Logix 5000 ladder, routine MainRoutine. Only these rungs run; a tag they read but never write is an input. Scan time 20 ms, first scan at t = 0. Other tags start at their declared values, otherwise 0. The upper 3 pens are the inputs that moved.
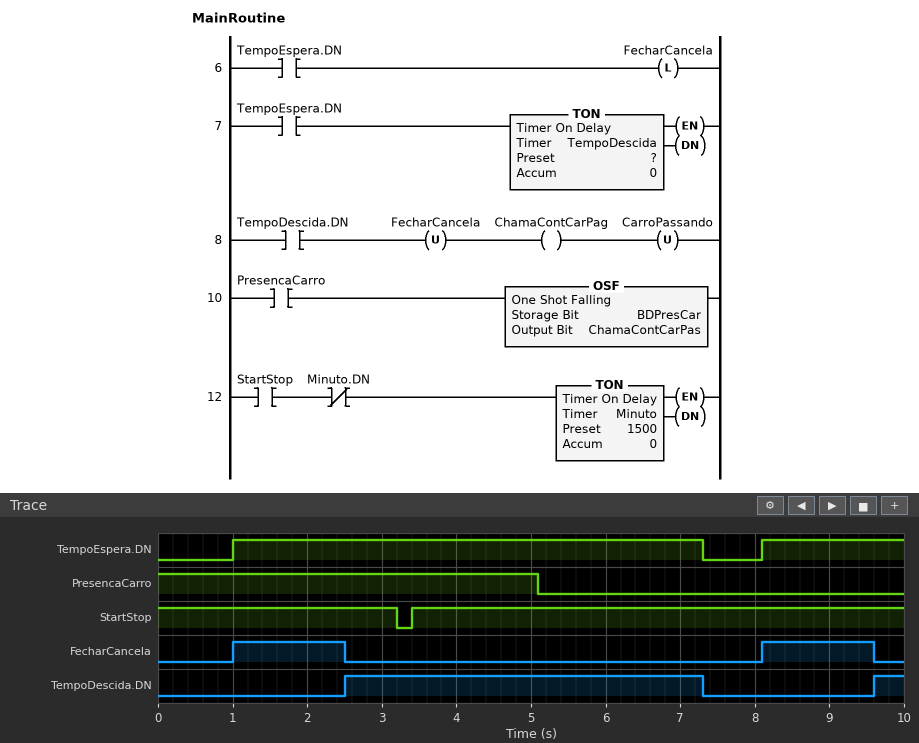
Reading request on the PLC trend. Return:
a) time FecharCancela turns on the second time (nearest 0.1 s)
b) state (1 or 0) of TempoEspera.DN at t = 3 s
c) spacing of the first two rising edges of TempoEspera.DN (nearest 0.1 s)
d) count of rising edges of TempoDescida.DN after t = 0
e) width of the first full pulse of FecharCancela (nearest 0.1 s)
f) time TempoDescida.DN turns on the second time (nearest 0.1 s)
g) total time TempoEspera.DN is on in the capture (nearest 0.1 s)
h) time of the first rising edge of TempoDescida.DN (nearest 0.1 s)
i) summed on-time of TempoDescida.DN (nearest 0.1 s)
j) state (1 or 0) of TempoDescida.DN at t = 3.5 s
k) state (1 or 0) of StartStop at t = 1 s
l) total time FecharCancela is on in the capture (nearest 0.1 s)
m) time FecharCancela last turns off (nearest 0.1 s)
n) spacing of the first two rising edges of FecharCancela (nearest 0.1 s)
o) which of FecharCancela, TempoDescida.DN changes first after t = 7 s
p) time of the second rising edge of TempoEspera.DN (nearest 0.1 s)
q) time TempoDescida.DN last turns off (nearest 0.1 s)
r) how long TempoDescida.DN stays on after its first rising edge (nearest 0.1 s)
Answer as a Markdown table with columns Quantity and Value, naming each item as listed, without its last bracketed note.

| Quantity | Value |
|---|---|
| time FecharCancela turns on the second time | 8.1 s |
| state (1 or 0) of TempoEspera.DN at t = 3 s | 1 |
| spacing of the first two rising edges of TempoEspera.DN | 7.1 s |
| count of rising edges of TempoDescida.DN after t = 0 | 2 |
| width of the first full pulse of FecharCancela | 1.5 s |
| time TempoDescida.DN turns on the second time | 9.6 s |
| total time TempoEspera.DN is on in the capture | 8.2 s |
| time of the first rising edge of TempoDescida.DN | 2.5 s |
| summed on-time of TempoDescida.DN | 5.2 s |
| state (1 or 0) of TempoDescida.DN at t = 3.5 s | 1 |
| state (1 or 0) of StartStop at t = 1 s | 1 |
| total time FecharCancela is on in the capture | 3.0 s |
| time FecharCancela last turns off | 9.6 s |
| spacing of the first two rising edges of FecharCancela | 7.1 s |
| which of FecharCancela, TempoDescida.DN changes first after t = 7 s | TempoDescida.DN |
| time of the second rising edge of TempoEspera.DN | 8.1 s |
| time TempoDescida.DN last turns off | 7.3 s |
| how long TempoDescida.DN stays on after its first rising edge | 4.8 s |
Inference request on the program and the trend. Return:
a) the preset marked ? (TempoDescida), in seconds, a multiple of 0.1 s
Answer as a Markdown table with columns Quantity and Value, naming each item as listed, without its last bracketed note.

| Quantity | Value |
|---|---|
| the preset marked ? (TempoDescida), in seconds, a multiple of 0.1 s | 1.5 s |
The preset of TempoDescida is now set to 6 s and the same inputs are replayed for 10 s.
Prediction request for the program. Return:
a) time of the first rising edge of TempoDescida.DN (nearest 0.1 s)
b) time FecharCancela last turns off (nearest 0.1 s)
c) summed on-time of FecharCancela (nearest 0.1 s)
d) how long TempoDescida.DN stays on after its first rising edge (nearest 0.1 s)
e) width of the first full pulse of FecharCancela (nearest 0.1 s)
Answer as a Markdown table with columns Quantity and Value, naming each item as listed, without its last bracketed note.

| Quantity | Value |
|---|---|
| time of the first rising edge of TempoDescida.DN | 7.0 s |
| time FecharCancela last turns off | 7.0 s |
| summed on-time of FecharCancela | 7.9 s |
| how long TempoDescida.DN stays on after its first rising edge | 0.3 s |
| width of the first full pulse of FecharCancela | 6.0 s |
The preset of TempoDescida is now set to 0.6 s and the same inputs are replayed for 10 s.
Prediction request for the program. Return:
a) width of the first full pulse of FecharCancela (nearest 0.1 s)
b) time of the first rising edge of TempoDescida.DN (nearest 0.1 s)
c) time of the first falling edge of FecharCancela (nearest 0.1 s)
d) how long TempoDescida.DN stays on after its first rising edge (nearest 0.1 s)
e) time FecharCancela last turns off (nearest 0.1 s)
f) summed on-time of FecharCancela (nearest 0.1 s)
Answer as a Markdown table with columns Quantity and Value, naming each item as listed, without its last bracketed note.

| Quantity | Value |
|---|---|
| width of the first full pulse of FecharCancela | 0.6 s |
| time of the first rising edge of TempoDescida.DN | 1.6 s |
| time of the first falling edge of FecharCancela | 1.6 s |
| how long TempoDescida.DN stays on after its first rising edge | 5.7 s |
| time FecharCancela last turns off | 8.7 s |
| summed on-time of FecharCancela | 1.2 s |
